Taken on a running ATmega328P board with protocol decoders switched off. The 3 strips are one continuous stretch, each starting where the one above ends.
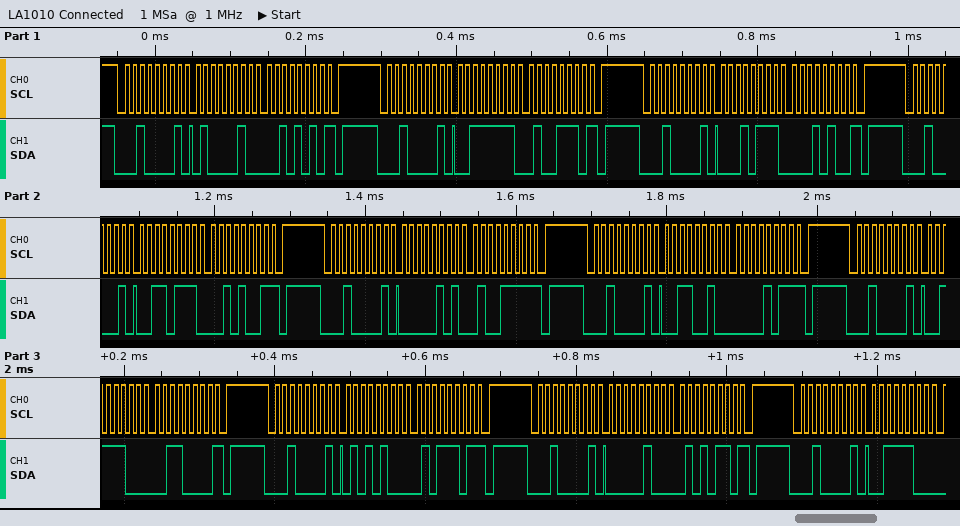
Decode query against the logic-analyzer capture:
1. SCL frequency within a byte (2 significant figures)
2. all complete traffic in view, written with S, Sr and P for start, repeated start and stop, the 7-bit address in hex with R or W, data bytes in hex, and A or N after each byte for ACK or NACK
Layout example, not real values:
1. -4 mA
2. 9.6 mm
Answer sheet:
1. 100 kHz
2. S 10R A 42 A 2A N P S 10R A 3F A 4E N P S 10R A 17 A 14 N P S 10R A 37 A 29 N P S 10R A 05 A 4F N P S 10R A 32 A 0B N P S 10R A 3C A 30 N P S 10R A 54 A 5D N P S 10R A 04 A 56 N P S 10R A 3C A
